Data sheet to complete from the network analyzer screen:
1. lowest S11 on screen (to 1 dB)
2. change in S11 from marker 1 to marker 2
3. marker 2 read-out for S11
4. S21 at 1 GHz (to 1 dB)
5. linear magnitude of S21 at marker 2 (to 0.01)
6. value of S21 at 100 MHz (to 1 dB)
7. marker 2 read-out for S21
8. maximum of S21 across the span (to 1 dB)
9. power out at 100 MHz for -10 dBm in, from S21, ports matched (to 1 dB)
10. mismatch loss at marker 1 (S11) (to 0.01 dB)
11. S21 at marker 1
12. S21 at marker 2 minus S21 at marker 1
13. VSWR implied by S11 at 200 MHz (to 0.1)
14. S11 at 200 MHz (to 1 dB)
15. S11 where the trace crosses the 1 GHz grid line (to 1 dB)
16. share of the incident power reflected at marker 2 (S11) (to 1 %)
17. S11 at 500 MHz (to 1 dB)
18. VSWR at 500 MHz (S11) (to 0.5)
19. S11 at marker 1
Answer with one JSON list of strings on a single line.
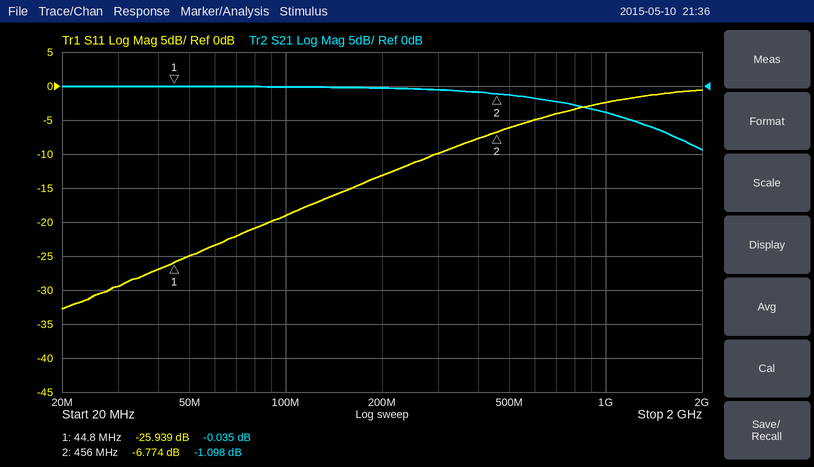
["-33 dB", "19.165 dB", "-6.774 dB", "-4 dB", "0.88", "0 dB", "-1.098 dB", "0 dB", "-10 dBm", "0.01 dB", "-0.035 dB", "-1.063 dB", "1.6", "-13 dB", "-2 dB", "21 %", "-6 dB", "3.0", "-25.939 dB"]
